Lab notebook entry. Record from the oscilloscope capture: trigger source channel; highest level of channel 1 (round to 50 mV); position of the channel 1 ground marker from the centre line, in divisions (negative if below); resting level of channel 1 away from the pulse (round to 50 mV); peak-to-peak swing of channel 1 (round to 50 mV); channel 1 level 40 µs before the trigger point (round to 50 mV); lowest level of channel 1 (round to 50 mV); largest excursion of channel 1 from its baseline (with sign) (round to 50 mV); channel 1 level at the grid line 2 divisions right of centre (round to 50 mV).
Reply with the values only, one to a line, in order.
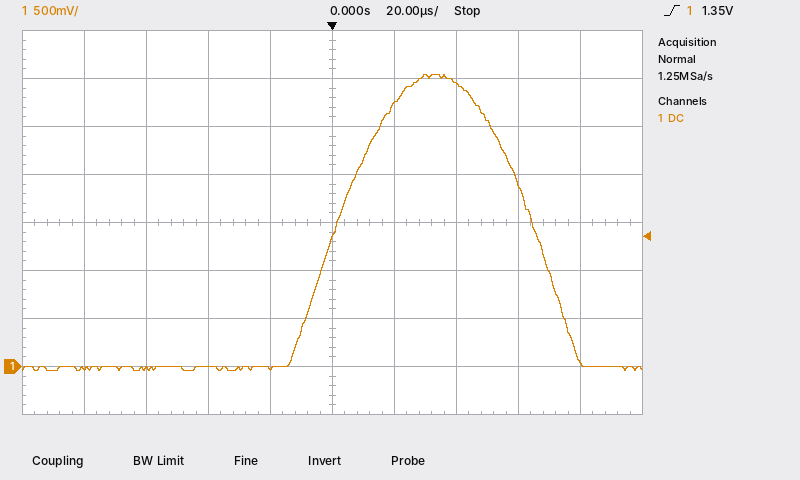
channel 1
3.05 V
-3.0 div
0 mV
3.10 V
0 mV
-50 mV
+3.05 V
2.95 V
